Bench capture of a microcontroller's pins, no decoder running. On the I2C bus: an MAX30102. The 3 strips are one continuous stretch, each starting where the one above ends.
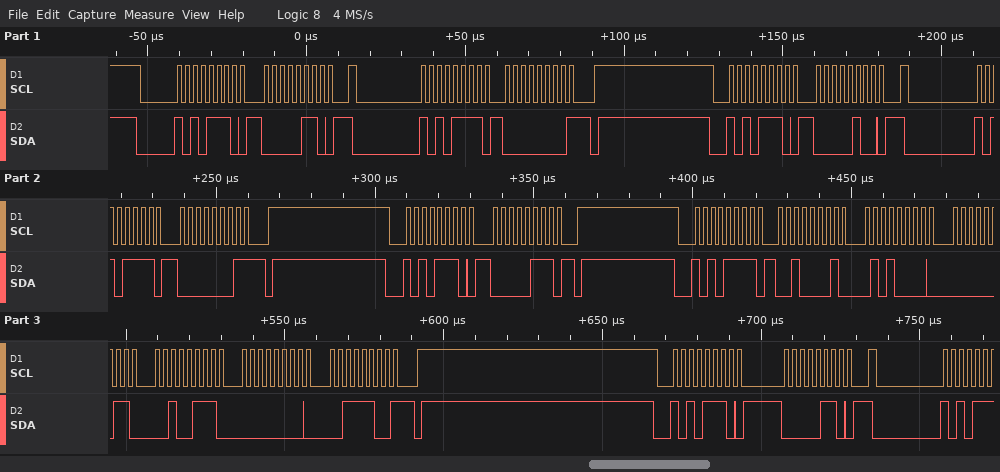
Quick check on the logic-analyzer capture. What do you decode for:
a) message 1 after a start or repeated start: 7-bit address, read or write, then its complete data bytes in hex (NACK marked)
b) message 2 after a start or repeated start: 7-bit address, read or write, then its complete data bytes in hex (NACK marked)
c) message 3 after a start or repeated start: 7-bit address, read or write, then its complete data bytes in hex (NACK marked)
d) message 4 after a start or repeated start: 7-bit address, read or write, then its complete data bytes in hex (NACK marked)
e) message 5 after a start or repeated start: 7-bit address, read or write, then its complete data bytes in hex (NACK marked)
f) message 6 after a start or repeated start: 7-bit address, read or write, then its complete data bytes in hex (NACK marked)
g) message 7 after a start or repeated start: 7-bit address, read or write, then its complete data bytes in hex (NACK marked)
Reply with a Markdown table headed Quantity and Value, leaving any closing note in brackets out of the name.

| Quantity | Value |
|---|---|
| message 1 after a start or repeated start: 7-bit address, read or write, then its complete data bytes in hex | 0x57 write: 06 |
| message 2 after a start or repeated start: 7-bit address, read or write, then its complete data bytes in hex | 0x57 read: 00 NACK |
| message 3 after a start or repeated start: 7-bit address, read or write, then its complete data bytes in hex | 0x57 write: 04 |
| message 4 after a start or repeated start: 7-bit address, read or write, then its complete data bytes in hex | 0x57 read: 01 NACK |
| message 5 after a start or repeated start: 7-bit address, read or write, then its complete data bytes in hex | 0x57 write: 07 |
| message 6 after a start or repeated start: 7-bit address, read or write, then its complete data bytes in hex | 0x57 read: 21 50 03 27 00 3C NACK |
| message 7 after a start or repeated start: 7-bit address, read or write, then its complete data bytes in hex | 0x57 write: 06 |
